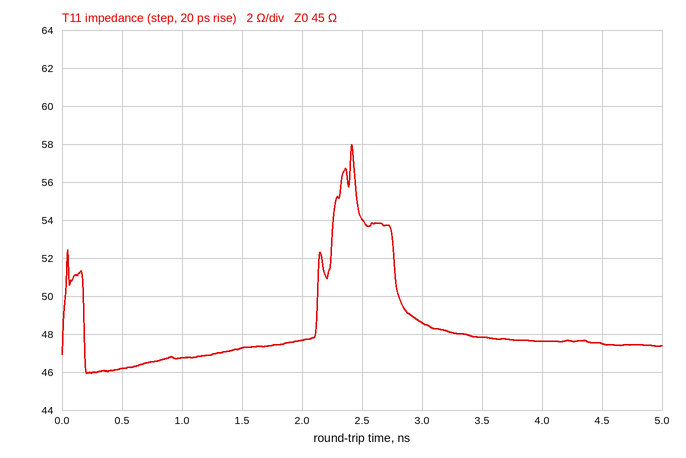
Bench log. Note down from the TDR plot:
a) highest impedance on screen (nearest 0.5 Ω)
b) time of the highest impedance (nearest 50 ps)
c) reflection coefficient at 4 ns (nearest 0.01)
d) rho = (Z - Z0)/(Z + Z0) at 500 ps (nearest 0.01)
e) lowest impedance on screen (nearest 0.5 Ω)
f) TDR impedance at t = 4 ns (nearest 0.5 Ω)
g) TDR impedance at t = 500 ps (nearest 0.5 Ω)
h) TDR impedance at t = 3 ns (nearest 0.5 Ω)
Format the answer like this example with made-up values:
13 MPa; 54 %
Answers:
58.0 Ω; 2.40 ns; +0.03; +0.01; 46.0 Ω; 47.5 Ω; 46.0 Ω; 48.5 Ω
